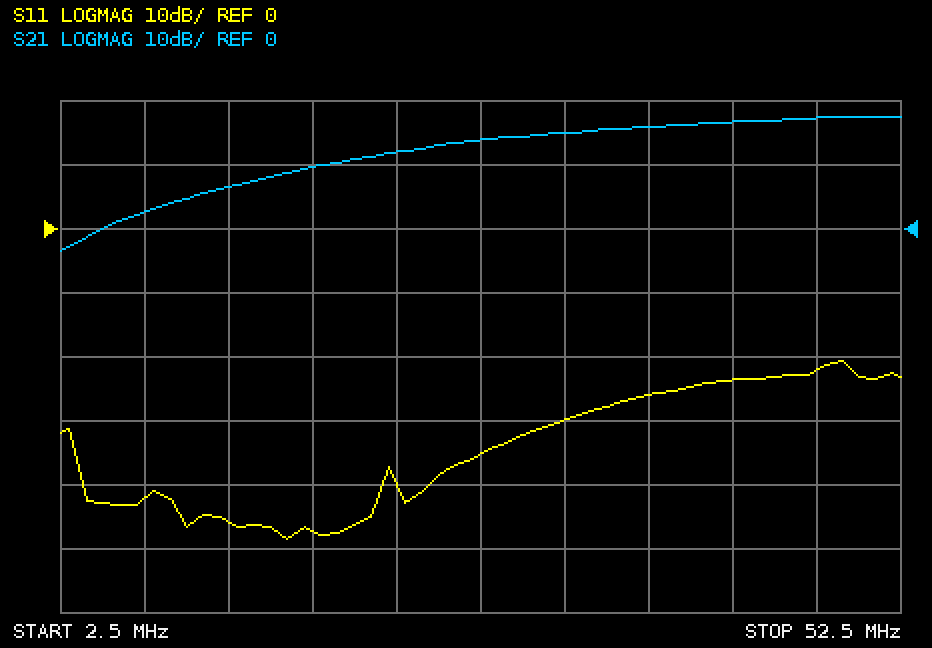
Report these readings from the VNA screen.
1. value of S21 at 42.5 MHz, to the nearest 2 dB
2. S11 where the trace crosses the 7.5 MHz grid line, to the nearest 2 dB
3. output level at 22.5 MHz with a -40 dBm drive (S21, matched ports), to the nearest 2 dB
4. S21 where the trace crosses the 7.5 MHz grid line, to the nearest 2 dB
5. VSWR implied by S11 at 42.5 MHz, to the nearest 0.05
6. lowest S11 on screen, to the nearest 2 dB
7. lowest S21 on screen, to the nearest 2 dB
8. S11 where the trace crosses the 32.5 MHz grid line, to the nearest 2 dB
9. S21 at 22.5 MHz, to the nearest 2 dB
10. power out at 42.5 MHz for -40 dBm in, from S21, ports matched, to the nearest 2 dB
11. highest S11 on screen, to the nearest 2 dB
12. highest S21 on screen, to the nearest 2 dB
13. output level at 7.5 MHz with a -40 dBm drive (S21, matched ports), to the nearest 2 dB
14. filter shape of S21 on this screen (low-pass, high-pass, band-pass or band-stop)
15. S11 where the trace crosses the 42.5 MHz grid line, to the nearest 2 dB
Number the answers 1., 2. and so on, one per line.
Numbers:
1. 16 dB
2. -42 dB
3. -28 dBm
4. 2 dB
5. 1.15
6. -48 dB
7. -4 dB
8. -30 dB
9. 12 dB
10. -24 dBm
11. -20 dB
12. 18 dB
13. -38 dBm
14. high-pass
15. -24 dB
